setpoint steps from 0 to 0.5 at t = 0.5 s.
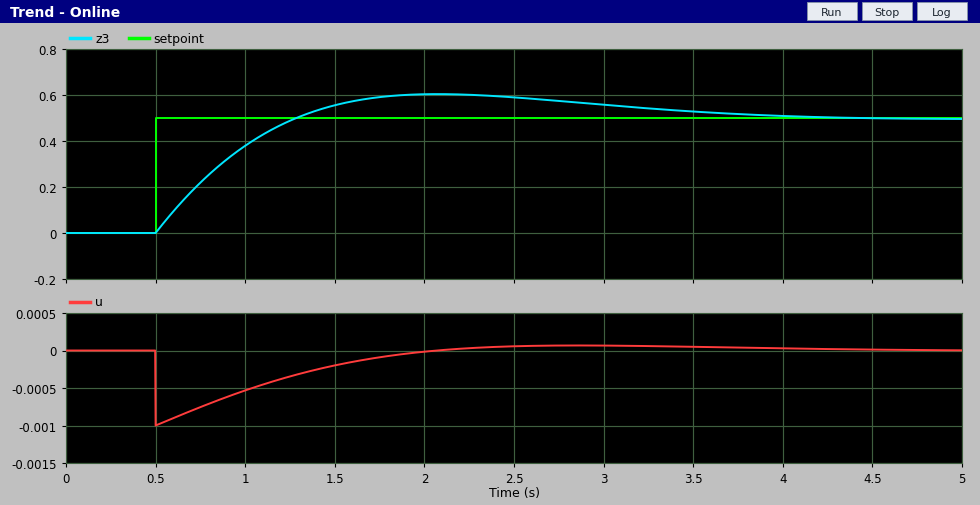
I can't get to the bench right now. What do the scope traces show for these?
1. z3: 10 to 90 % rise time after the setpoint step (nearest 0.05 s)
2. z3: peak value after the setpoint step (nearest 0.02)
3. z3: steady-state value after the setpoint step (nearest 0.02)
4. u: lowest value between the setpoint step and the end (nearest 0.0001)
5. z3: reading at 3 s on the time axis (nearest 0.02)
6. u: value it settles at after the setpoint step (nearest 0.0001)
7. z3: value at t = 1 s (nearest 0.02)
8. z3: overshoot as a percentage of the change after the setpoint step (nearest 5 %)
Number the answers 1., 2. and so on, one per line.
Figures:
1. 0.60 s
2. 0.60
3. 0.50
4. -0.0010
5. 0.56
6. 0.0000
7. 0.38
8. 20 %
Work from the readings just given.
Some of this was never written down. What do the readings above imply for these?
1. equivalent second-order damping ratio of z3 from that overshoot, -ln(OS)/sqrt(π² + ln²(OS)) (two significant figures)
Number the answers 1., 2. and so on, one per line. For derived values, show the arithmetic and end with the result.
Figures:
1. ln(0.2) = -1.609; 1.609 / sqrt(9.870 + 2.590) = 0.46
